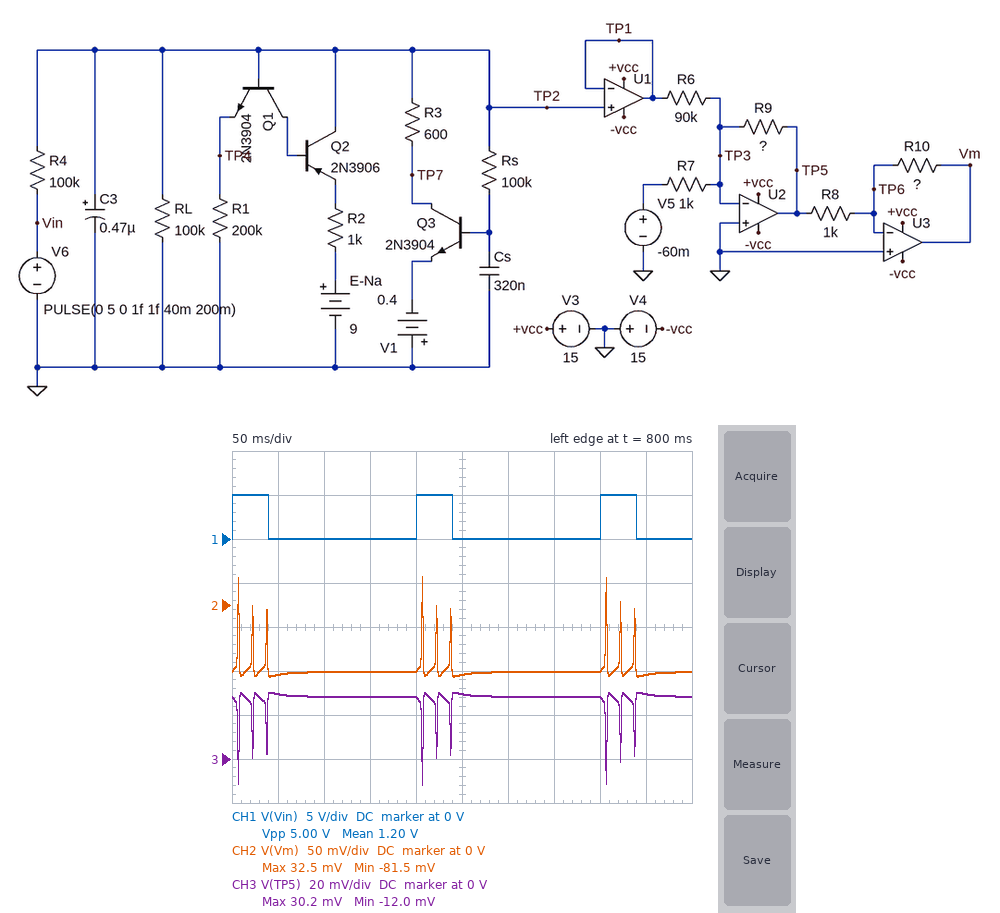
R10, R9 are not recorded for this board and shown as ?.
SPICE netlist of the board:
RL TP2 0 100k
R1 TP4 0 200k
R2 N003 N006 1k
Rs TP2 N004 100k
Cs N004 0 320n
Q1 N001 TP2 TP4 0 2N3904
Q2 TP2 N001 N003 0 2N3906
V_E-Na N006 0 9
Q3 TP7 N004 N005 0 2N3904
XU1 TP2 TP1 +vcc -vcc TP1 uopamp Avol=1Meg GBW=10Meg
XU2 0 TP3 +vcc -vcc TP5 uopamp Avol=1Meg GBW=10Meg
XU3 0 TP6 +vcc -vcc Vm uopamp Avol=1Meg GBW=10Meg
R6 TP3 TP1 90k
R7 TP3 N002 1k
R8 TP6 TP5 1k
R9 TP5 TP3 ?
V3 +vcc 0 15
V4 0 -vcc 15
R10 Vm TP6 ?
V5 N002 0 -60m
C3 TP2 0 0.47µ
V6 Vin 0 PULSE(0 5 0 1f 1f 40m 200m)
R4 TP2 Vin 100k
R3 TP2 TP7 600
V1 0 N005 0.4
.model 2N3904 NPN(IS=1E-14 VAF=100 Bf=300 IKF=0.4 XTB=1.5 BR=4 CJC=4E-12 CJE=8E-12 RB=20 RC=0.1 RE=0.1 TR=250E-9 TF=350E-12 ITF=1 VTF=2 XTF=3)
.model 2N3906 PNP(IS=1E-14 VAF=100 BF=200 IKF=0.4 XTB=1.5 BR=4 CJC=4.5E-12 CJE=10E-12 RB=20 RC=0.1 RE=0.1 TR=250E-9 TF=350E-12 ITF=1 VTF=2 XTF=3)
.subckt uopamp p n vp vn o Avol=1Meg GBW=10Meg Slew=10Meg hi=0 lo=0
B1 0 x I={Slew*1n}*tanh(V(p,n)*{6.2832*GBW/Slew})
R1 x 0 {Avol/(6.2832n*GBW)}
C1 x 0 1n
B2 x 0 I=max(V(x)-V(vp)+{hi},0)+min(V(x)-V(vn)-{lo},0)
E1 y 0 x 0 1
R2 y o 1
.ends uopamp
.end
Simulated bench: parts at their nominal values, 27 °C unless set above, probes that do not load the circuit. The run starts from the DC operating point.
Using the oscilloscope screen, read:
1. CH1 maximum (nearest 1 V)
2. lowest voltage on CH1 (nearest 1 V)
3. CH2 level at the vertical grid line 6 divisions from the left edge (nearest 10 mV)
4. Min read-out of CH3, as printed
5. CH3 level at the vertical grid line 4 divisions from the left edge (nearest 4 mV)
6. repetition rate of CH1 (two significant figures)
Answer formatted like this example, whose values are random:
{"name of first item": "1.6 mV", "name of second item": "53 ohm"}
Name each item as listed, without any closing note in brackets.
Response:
{"CH1 maximum": "5 V", "lowest voltage on CH1": "0 V", "CH2 level at the vertical grid line 6 divisions from the left edge": "-80 mV", "Min read-out of CH3, as printed": "-12.0 mV", "CH3 level at the vertical grid line 4 divisions from the left edge": "28 mV", "repetition rate of CH1": "5.0 Hz"}
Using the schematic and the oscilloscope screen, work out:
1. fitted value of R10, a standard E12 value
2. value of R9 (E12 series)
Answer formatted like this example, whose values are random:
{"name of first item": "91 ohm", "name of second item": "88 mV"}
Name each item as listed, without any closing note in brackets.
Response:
{"fitted value of R10, a standard E12 value": "2.7 kΩ", "value of R9": "470 Ω"}
